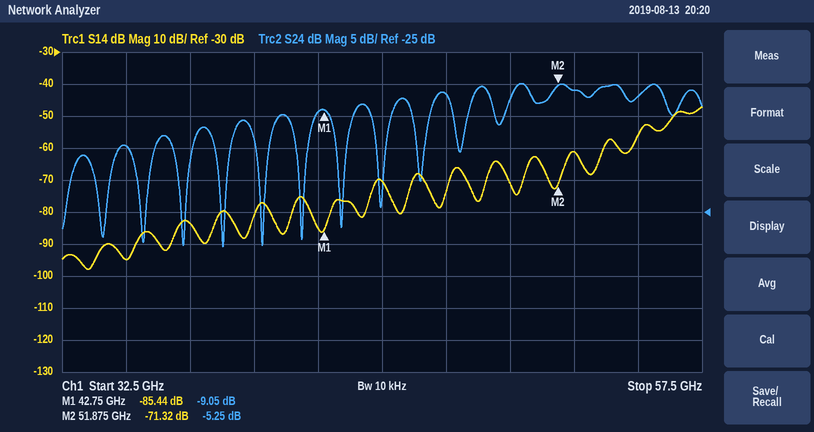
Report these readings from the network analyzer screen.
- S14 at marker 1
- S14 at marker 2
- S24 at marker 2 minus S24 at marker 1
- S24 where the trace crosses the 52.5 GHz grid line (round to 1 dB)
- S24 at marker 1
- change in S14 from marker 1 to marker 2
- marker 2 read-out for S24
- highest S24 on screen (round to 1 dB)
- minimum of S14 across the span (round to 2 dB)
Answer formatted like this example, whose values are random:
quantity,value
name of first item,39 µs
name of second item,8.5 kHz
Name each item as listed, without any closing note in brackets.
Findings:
quantity,value
S14 at marker 1,-85.44 dB
S14 at marker 2,-71.32 dB
S24 at marker 2 minus S24 at marker 1,3.80 dB
S24 where the trace crosses the 52.5 GHz grid line,-6 dB
S24 at marker 1,-9.05 dB
change in S14 from marker 1 to marker 2,14.12 dB
marker 2 read-out for S24,-5.25 dB
highest S24 on screen,-5 dB
minimum of S14 across the span,-98 dB
